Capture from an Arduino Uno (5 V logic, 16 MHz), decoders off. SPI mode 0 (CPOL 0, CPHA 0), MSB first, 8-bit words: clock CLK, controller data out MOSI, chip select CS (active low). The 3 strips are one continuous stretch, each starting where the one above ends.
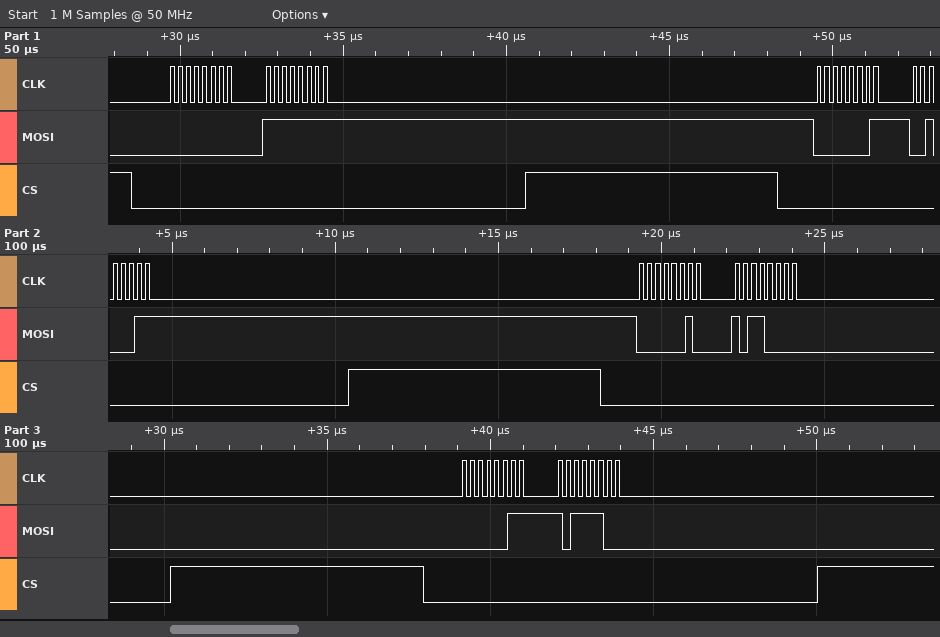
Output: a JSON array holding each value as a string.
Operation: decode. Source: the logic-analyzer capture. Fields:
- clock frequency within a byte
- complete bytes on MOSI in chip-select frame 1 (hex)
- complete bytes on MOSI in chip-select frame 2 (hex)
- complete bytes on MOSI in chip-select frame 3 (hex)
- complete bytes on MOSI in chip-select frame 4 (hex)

["4 MHz", "00 FF", "01 23", "02 B0", "03 BC"]
